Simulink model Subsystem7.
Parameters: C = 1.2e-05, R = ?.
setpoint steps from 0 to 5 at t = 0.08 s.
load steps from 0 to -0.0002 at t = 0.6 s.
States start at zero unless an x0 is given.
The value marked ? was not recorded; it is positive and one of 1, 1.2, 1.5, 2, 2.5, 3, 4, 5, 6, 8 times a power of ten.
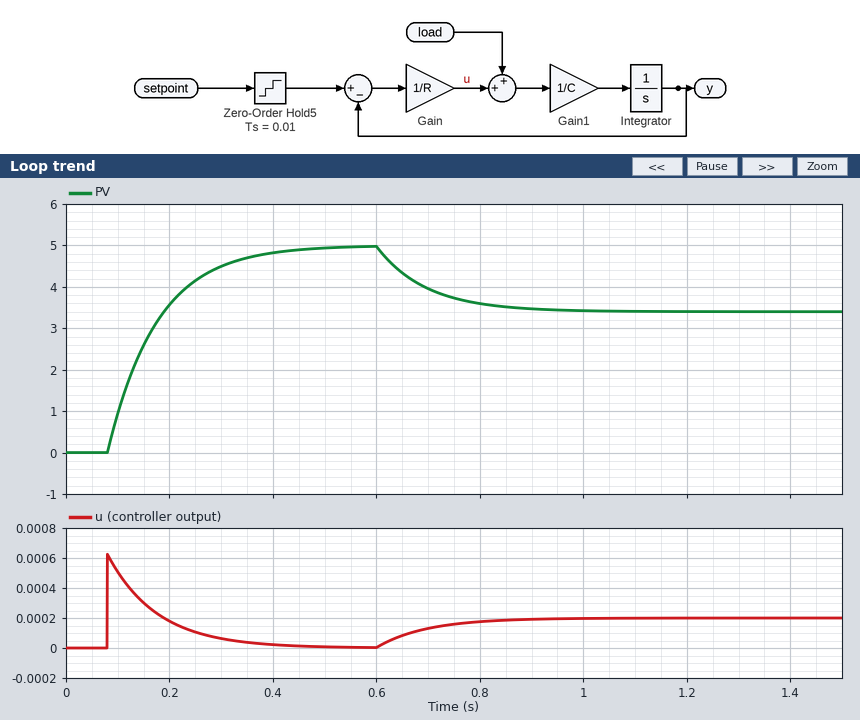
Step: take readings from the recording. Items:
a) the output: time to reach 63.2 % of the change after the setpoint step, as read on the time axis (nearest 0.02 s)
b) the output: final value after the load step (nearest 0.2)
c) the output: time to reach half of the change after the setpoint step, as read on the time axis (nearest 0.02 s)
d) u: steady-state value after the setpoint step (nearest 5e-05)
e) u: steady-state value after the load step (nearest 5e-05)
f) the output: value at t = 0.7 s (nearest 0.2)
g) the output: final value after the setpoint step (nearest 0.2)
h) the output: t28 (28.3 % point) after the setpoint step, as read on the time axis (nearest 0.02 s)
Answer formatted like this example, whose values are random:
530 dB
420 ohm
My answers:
0.18 s
3.4
0.14 s
0.00000
0.00020
4.0
5.0
0.12 s
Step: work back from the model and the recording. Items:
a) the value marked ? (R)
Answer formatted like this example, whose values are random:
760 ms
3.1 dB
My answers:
8000
